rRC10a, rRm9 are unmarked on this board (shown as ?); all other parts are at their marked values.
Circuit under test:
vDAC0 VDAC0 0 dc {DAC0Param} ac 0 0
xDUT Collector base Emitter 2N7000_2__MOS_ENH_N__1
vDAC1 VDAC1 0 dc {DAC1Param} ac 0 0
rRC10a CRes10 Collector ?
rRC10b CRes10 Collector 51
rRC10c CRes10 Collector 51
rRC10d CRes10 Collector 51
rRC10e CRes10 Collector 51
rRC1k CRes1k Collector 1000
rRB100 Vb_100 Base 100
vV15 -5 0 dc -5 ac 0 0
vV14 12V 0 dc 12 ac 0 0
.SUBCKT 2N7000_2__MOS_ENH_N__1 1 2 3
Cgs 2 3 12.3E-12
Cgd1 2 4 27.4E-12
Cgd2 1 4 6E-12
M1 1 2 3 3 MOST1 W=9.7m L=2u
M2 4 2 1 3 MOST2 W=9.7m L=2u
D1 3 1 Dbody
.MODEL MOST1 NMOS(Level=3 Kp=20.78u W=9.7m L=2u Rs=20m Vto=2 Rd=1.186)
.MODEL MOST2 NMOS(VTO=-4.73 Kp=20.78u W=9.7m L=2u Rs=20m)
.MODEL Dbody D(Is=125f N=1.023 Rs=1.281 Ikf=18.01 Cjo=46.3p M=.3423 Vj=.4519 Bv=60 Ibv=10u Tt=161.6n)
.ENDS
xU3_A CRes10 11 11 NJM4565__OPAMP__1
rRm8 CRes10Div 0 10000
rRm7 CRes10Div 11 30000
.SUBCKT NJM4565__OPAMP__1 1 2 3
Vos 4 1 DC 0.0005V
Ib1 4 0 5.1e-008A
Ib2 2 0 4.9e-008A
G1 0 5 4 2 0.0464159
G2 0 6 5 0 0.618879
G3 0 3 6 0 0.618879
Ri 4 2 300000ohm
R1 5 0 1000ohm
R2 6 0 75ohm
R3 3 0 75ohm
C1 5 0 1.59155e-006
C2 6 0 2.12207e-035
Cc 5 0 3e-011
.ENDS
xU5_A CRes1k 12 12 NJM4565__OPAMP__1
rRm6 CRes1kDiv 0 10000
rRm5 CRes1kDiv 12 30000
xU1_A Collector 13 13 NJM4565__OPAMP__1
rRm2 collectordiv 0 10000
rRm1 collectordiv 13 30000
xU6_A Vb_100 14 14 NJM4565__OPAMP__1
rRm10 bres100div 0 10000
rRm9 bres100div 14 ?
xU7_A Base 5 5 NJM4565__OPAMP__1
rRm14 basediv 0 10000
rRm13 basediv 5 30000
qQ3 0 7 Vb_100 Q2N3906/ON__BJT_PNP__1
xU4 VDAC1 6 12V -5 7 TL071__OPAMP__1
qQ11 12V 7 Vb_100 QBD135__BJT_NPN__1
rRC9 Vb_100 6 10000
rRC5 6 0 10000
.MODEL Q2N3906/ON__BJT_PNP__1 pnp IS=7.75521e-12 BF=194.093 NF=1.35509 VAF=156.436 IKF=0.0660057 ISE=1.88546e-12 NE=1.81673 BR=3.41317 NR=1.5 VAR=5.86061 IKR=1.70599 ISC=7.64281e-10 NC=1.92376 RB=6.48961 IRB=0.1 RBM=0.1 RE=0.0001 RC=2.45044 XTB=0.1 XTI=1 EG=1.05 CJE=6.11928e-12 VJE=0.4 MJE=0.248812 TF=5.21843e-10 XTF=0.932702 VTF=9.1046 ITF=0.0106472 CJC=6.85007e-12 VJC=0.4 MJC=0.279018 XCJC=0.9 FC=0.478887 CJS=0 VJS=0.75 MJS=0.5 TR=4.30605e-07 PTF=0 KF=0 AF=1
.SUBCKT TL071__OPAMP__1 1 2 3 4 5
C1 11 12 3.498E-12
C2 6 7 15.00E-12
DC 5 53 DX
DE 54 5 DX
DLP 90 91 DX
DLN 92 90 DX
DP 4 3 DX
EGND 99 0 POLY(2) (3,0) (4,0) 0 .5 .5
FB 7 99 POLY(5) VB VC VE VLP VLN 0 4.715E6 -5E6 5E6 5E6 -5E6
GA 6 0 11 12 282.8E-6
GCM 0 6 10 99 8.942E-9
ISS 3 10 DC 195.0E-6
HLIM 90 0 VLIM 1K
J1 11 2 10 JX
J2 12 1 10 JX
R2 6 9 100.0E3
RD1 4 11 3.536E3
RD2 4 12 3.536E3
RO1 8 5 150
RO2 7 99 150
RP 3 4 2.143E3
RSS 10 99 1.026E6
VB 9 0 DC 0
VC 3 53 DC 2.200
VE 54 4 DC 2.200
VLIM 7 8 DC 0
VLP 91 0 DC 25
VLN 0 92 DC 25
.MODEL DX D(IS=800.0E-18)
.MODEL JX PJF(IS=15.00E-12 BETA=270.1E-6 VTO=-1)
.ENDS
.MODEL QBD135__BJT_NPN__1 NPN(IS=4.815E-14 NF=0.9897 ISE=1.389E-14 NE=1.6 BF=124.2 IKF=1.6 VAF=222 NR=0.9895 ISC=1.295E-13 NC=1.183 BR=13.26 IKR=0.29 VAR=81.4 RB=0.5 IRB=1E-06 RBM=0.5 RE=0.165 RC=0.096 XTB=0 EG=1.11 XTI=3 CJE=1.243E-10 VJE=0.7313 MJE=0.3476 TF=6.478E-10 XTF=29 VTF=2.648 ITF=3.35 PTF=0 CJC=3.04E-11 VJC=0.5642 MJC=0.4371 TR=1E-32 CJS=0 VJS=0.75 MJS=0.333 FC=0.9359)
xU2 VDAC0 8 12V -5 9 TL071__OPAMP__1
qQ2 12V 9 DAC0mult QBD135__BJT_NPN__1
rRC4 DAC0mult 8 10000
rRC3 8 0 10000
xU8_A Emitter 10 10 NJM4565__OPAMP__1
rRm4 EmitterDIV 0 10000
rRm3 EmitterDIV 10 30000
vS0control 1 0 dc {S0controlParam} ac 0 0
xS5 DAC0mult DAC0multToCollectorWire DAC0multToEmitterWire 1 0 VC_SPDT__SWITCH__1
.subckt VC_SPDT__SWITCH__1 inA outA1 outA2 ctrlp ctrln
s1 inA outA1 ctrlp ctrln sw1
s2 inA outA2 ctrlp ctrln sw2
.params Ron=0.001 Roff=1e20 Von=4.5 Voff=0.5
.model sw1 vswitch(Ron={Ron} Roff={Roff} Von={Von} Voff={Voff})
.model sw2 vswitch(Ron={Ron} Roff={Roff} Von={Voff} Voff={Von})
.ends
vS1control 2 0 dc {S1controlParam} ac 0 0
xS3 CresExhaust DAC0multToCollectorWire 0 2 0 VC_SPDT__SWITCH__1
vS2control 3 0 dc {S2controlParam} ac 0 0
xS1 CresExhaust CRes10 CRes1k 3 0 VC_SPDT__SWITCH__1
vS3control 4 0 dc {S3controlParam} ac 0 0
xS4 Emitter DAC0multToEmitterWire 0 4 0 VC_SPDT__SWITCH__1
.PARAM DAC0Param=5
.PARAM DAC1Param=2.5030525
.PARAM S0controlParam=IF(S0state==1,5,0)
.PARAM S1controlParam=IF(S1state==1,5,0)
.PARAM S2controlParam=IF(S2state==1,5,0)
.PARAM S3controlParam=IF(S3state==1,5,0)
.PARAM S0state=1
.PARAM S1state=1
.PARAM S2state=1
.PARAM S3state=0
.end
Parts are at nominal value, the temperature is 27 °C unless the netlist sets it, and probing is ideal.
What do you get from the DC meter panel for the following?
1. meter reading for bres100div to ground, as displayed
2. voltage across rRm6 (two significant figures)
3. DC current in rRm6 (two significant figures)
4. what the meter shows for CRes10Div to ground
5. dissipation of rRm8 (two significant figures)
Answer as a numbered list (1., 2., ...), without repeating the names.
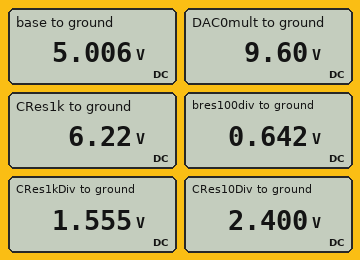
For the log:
1. 0.642 V
2. 1.6 V
3. 160 µA
4. 2.400 V
5. 580 µW
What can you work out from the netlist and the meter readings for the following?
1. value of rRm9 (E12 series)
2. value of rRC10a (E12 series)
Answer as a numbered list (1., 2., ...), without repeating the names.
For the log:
1. 68 kΩ
2. 18 Ω
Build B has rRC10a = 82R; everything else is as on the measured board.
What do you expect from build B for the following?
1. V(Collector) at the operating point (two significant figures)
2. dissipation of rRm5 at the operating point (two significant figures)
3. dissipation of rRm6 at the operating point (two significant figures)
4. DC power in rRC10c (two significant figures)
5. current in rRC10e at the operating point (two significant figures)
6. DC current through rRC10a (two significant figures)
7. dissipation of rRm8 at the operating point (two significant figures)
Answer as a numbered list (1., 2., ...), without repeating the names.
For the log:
1. 4.6 V
2. 400 µW
3. 130 µW
4. 490 mW
5. 98 mA
6. 61 mA
7. 580 µW
